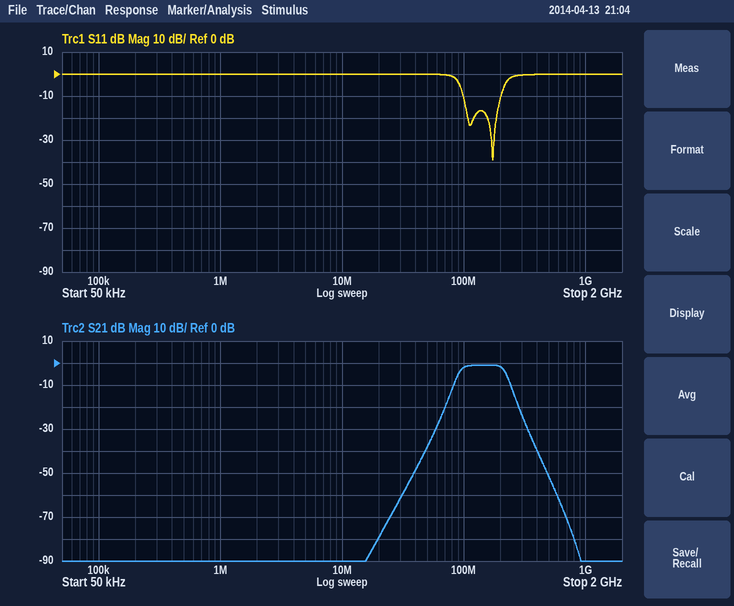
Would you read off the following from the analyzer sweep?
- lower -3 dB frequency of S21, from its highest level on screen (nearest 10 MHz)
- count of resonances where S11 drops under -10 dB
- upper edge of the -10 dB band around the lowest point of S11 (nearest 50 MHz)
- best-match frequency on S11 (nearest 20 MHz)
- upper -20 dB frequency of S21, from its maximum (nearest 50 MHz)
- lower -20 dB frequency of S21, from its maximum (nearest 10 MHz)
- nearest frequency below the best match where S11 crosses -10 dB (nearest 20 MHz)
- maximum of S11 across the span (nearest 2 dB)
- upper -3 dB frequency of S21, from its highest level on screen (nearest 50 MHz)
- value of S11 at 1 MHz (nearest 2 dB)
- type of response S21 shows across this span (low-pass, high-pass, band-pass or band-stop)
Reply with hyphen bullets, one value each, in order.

- 90 MHz
- 2
- 200 MHz
- 180 MHz
- 300 MHz
- 70 MHz
- 100 MHz
- 0 dB
- 200 MHz
- 0 dB
- band-pass
